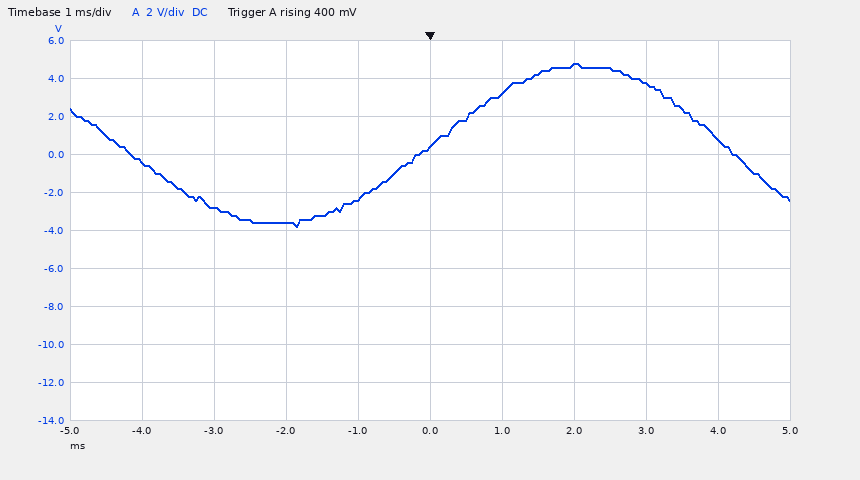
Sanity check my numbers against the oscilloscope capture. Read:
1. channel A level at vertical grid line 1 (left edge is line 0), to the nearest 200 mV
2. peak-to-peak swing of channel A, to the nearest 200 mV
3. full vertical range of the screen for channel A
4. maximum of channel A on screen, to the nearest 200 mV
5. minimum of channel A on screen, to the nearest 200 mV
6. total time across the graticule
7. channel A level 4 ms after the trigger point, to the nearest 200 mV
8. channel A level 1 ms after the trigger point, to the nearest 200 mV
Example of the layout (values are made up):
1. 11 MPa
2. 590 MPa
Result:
1. -400 mV
2. 8.6 V
3. 20 V
4. 4.8 V
5. -3.8 V
6. 10 ms
7. 800 mV
8. 3.2 V
